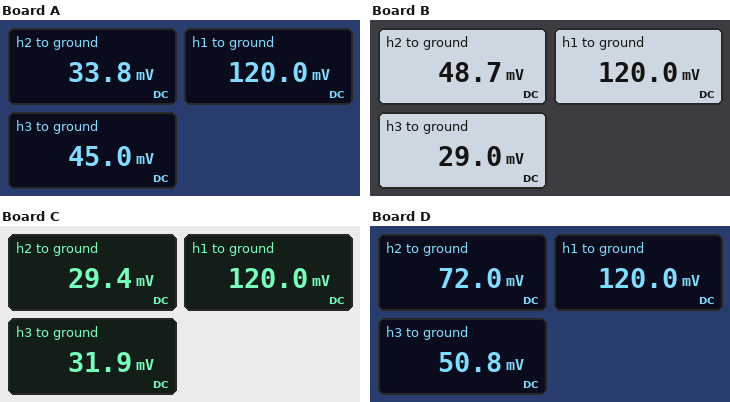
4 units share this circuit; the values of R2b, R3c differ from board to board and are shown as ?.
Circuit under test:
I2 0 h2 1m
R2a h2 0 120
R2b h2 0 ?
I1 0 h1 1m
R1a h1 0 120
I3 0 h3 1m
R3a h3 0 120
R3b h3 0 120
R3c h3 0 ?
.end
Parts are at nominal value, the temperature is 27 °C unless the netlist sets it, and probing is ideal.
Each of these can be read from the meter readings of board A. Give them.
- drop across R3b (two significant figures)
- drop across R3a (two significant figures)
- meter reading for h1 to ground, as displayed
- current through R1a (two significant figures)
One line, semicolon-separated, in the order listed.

45 mV; 45 mV; 120.0 mV; 1.0 mA
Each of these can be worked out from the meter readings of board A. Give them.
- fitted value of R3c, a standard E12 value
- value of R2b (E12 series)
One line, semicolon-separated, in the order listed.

180 Ω; 47 Ω
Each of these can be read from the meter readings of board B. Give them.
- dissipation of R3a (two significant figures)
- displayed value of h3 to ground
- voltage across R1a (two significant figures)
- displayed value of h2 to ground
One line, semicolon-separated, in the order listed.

7.0 µW; 29.0 mV; 120 mV; 48.7 mV
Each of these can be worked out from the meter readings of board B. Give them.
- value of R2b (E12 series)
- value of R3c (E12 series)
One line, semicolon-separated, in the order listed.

82 Ω; 56 Ω
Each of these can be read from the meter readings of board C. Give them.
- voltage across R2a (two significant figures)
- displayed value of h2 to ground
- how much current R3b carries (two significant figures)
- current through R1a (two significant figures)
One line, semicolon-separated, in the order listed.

29 mV; 29.4 mV; 270 µA; 1.0 mA
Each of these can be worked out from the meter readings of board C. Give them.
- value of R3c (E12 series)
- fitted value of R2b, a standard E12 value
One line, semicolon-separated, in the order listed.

68 Ω; 39 Ω
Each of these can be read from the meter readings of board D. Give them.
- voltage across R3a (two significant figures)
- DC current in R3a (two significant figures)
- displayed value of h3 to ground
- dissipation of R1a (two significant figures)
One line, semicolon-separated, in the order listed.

51 mV; 420 µA; 50.8 mV; 120 µW
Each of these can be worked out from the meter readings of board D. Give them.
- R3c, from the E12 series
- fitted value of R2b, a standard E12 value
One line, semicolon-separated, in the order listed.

330 Ω; 180 Ω
